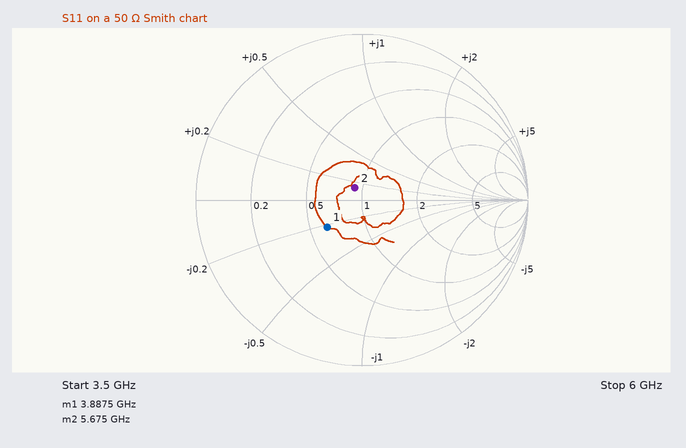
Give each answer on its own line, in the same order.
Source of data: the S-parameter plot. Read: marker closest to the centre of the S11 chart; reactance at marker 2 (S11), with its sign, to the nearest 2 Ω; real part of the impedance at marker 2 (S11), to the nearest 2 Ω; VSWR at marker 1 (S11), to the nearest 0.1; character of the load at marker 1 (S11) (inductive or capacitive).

marker 2
+6 Ω
46 Ω
1.7
capacitive
